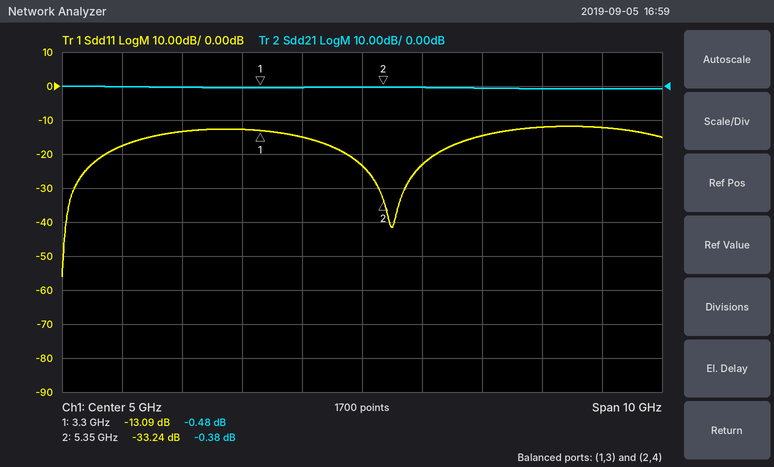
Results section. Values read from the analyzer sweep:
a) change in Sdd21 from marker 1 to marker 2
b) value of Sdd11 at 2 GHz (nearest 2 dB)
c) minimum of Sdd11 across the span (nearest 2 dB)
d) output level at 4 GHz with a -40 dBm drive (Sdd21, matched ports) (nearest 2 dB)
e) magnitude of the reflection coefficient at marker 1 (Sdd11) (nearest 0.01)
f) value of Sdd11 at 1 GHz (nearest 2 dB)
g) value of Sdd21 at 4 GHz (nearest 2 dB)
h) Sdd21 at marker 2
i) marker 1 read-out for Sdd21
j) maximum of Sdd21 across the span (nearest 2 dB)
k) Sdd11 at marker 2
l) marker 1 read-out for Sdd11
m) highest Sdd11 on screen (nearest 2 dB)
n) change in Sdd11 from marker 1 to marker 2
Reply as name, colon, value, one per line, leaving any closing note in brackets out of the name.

change in Sdd21 from marker 1 to marker 2: 0.10 dB
value of Sdd11 at 2 GHz: -14 dB
minimum of Sdd11 across the span: -56 dB
output level at 4 GHz with a -40 dBm drive (Sdd21, matched ports): -40 dBm
magnitude of the reflection coefficient at marker 1 (Sdd11): 0.22
value of Sdd11 at 1 GHz: -18 dB
value of Sdd21 at 4 GHz: 0 dB
Sdd21 at marker 2: -0.38 dB
marker 1 read-out for Sdd21: -0.48 dB
maximum of Sdd21 across the span: 0 dB
Sdd11 at marker 2: -33.24 dB
marker 1 read-out for Sdd11: -13.09 dB
highest Sdd11 on screen: -12 dB
change in Sdd11 from marker 1 to marker 2: -20.15 dB
